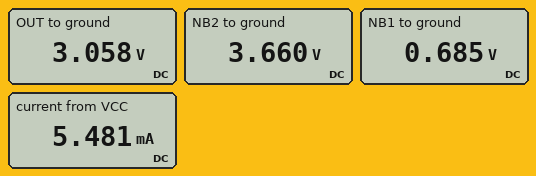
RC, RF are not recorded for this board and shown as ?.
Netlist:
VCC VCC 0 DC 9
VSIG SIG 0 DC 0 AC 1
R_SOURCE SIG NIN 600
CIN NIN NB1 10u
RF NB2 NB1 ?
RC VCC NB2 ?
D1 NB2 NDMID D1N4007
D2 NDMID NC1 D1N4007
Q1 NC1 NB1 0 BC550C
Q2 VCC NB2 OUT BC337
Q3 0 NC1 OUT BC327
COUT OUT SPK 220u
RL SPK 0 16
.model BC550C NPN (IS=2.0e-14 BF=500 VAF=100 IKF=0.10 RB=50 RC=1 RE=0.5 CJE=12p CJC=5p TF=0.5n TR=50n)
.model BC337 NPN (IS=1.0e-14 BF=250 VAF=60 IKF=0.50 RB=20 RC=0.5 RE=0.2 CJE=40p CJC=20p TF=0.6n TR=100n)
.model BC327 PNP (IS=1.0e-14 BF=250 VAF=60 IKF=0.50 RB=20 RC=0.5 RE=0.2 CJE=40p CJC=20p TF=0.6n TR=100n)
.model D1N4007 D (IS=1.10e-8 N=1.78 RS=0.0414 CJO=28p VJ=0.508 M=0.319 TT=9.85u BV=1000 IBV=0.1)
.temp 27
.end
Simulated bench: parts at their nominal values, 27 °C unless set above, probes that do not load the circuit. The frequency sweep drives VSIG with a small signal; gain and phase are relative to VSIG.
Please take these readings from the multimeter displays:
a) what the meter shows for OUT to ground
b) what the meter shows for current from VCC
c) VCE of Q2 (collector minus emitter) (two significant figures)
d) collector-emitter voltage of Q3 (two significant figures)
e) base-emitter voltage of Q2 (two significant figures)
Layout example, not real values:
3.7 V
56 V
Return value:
3.058 V
5.481 mA
5.9 V
-3.1 V
600 mV
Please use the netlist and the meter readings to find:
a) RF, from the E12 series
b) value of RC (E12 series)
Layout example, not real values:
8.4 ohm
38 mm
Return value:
270 kΩ
1 kΩ
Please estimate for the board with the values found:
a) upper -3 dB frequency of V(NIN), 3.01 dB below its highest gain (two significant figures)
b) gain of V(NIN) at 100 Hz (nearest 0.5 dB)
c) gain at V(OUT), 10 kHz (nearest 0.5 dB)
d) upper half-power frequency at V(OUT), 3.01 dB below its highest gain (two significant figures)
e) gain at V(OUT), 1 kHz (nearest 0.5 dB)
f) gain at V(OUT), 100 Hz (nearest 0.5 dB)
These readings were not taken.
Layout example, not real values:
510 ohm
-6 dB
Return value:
21 Hz
-4.0 dB
23.5 dB
22 Hz
23.5 dB
24.5 dB
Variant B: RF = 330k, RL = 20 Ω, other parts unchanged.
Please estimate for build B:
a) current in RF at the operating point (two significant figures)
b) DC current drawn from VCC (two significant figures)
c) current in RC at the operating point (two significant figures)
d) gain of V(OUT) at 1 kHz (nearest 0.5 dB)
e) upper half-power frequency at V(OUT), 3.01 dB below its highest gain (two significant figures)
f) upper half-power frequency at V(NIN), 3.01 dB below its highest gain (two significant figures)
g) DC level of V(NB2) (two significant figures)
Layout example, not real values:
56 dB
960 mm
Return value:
10 µA
5.1 mA
5.0 mA
24.5 dB
20 Hz
27 Hz
4.0 V
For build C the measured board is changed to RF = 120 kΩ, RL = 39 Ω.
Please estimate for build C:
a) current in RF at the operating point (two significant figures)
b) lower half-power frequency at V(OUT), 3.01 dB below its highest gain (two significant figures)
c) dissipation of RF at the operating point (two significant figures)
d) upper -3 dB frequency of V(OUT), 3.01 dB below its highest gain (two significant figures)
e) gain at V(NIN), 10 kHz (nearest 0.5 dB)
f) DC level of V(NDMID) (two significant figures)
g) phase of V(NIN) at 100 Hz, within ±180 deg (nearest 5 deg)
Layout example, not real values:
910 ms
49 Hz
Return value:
14 µA
5.2 Hz
24 µW
460 kHz
-7.0 dB
1.8 V
-10 deg
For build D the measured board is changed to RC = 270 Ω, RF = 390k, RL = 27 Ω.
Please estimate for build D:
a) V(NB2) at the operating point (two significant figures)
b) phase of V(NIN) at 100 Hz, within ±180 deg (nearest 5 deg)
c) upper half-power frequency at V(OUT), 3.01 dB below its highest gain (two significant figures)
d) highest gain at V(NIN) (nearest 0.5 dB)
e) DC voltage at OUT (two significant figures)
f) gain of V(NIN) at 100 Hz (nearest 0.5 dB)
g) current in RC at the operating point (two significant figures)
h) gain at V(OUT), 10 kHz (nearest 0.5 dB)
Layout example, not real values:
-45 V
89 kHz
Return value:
6.9 V
0 deg
40 Hz
0 dB
6.3 V
-3.0 dB
7.8 mA
24.5 dB
